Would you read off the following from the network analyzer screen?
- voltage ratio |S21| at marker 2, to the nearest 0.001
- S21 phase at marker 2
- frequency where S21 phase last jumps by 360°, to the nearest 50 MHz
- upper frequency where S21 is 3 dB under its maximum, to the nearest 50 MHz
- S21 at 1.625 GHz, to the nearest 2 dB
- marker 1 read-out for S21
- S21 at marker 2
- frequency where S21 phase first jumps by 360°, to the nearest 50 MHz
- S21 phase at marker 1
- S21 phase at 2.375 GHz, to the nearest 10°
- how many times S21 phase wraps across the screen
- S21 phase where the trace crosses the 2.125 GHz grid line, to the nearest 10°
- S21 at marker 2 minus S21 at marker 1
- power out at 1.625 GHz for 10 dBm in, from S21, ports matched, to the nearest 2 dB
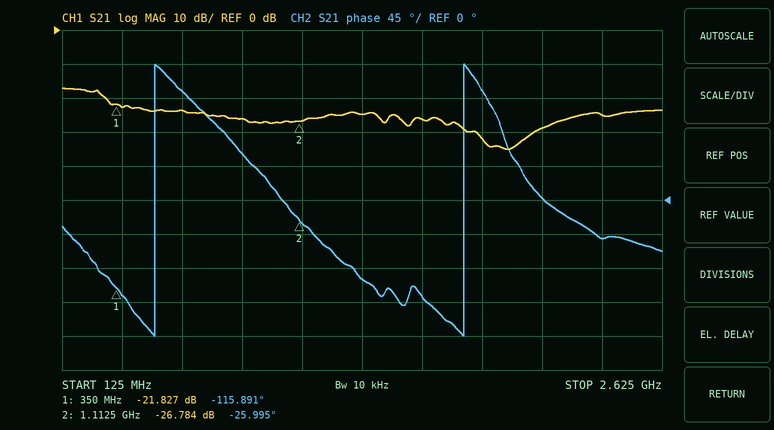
0.046
-25.995°
1.80 GHz
300 MHz
-26 dB
-21.827 dB
-26.784 dB
500 MHz
-115.891°
-50°
2
0°
-4.957 dB
-16 dBm
